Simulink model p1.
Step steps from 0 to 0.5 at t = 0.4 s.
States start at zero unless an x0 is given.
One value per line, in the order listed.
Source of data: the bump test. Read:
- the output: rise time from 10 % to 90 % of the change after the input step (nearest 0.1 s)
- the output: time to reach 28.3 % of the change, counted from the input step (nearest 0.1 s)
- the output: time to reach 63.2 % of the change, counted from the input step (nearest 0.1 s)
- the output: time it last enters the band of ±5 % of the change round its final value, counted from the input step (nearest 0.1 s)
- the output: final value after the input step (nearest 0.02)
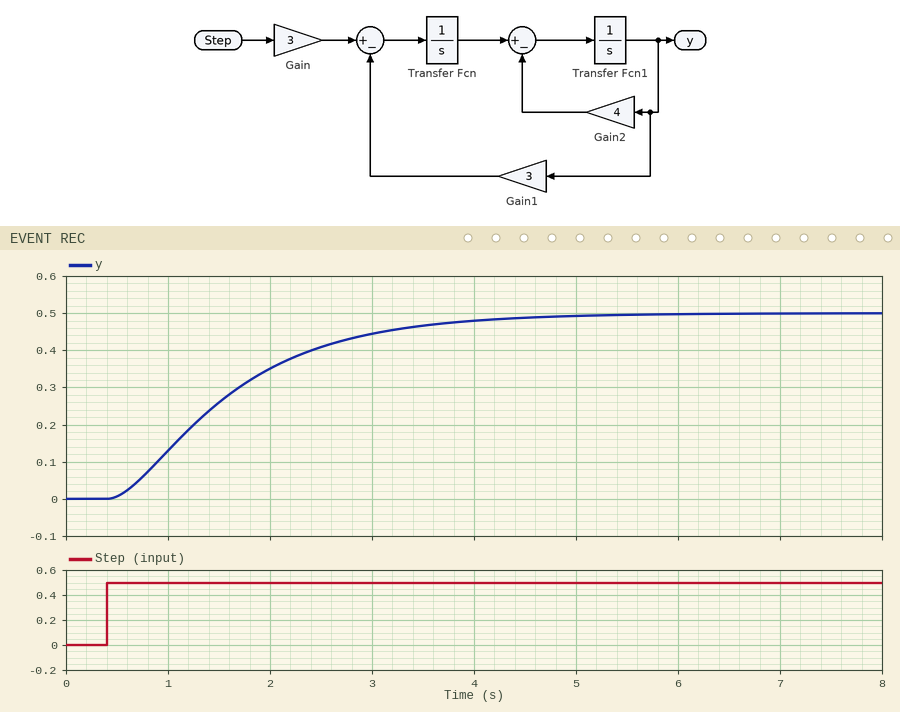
2.4 s
0.6 s
1.4 s
3.4 s
0.50
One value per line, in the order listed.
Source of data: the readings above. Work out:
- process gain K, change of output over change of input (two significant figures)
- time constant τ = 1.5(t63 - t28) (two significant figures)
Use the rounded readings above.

1.0
1.2 s
